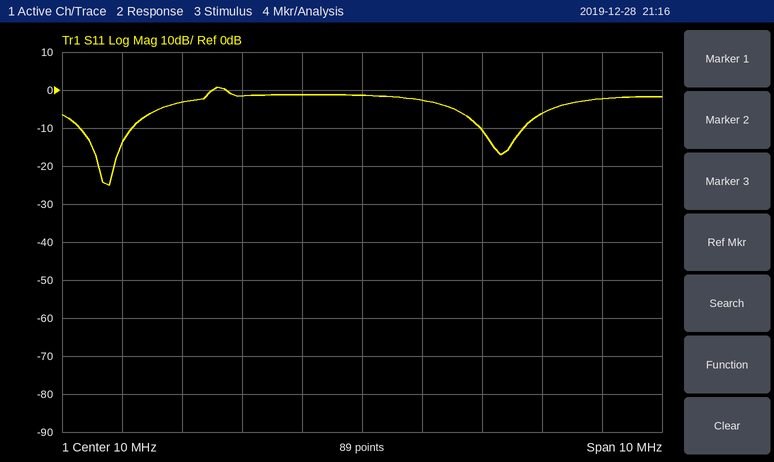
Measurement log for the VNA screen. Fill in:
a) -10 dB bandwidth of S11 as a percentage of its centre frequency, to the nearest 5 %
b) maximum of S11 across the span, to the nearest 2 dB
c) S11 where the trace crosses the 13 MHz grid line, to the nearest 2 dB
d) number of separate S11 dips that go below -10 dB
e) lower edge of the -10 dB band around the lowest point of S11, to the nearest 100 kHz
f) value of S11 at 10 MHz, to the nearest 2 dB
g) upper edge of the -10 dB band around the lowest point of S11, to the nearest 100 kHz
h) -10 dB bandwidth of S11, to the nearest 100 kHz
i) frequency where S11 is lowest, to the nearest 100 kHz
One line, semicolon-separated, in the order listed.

15 %; 0 dB; -6 dB; 2; 5.3 MHz; -2 dB; 6.2 MHz; 900 kHz; 5.8 MHz
